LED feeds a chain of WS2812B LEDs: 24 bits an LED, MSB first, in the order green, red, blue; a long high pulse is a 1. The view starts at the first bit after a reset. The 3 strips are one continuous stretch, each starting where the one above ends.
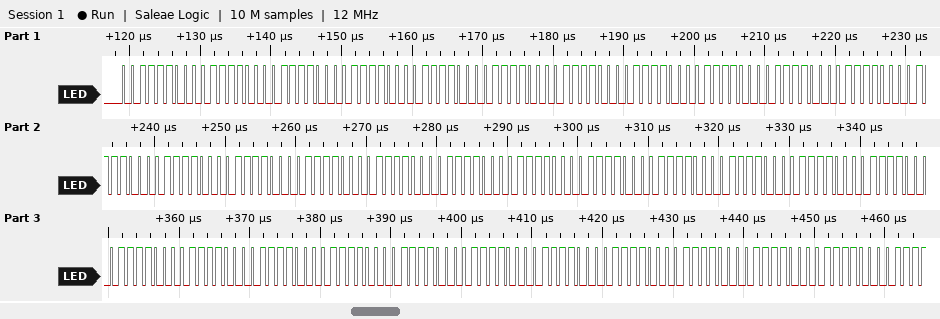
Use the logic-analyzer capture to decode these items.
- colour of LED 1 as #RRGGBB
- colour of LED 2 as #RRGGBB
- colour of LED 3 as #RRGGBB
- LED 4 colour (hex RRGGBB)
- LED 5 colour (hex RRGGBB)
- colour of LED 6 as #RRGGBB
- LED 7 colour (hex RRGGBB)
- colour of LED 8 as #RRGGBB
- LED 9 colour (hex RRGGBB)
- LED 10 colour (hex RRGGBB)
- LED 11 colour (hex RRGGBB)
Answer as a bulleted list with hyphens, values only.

- #3C3C3C
- #3C3C3C
- #3C3C3C
- #3C3C3C
- #3C3C3C
- #3C3C3C
- #3C3C3C
- #3C3C3C
- #3C3C3C
- #3C3C3C
- #3C3C3C
